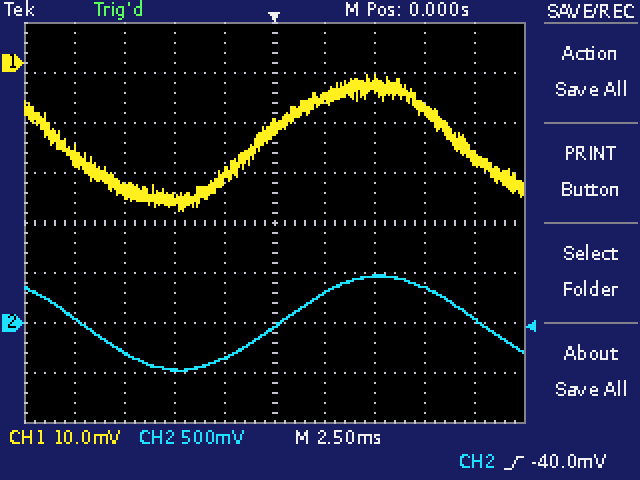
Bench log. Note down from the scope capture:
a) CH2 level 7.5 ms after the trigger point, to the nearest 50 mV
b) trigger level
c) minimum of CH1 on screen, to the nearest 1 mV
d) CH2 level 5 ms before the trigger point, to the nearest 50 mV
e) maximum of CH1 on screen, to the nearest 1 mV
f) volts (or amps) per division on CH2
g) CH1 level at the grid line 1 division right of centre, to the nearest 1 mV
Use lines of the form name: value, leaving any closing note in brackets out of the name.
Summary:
CH2 level 7.5 ms after the trigger point, to the nearest 50 mV: 350 mV
trigger level: -40.0 mV
minimum of CH1 on screen, to the nearest 1 mV: -30 mV
CH2 level 5 ms before the trigger point, to the nearest 50 mV: -450 mV
maximum of CH1 on screen, to the nearest 1 mV: -2 mV
volts (or amps) per division on CH2: 500 mV
CH1 level at the grid line 1 division right of centre, to the nearest 1 mV: -7 mV
